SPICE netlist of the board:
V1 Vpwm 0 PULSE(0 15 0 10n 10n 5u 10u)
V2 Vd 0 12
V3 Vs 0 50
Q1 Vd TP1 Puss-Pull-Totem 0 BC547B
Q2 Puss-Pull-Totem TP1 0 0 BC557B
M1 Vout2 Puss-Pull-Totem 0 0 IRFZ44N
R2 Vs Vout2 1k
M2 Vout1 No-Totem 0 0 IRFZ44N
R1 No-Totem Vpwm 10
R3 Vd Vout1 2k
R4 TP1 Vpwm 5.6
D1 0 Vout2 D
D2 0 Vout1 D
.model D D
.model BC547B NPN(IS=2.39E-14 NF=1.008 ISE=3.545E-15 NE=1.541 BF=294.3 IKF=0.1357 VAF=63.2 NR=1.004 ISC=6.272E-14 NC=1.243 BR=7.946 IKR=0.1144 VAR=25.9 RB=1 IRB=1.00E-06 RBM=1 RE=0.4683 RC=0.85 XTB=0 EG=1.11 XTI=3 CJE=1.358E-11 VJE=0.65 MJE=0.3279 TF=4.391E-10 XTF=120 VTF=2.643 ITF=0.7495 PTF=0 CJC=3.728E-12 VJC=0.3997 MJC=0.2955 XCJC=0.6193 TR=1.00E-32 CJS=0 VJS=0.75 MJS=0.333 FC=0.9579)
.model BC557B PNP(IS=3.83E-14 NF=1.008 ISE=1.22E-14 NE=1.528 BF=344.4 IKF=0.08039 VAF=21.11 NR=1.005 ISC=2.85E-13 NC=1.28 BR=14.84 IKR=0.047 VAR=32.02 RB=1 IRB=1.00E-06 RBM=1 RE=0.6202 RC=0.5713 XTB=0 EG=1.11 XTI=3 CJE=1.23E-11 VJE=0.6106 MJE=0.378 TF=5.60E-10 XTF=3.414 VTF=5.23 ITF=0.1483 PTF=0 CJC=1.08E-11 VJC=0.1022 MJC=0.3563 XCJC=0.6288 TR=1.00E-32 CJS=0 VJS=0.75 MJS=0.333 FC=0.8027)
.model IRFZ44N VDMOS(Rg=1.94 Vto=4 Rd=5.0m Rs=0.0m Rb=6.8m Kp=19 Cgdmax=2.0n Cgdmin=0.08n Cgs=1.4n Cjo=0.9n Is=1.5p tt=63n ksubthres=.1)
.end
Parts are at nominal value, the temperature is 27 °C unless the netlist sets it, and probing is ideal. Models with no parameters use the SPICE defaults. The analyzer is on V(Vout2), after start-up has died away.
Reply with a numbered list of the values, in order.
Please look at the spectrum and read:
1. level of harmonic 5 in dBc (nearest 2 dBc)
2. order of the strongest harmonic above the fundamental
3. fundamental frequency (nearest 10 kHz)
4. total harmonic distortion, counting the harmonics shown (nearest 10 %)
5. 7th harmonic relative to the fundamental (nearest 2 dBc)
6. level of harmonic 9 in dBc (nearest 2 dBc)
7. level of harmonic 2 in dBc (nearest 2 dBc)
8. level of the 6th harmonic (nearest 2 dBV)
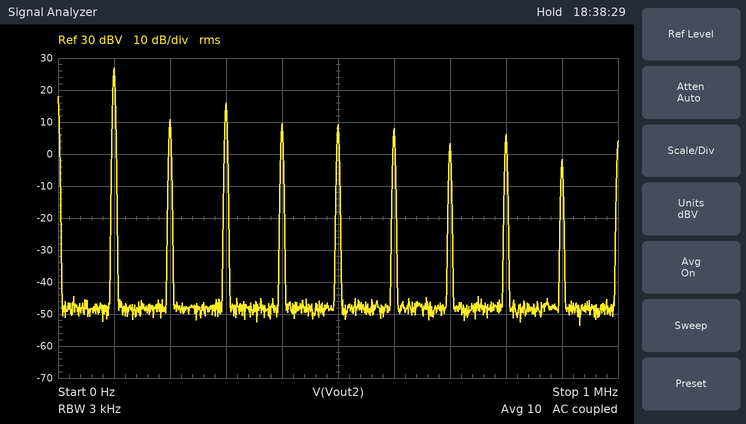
1. -18 dBc
2. 3
3. 100 kHz
4. 40 %
5. -24 dBc
6. -28 dBc
7. -16 dBc
8. 8 dBV
